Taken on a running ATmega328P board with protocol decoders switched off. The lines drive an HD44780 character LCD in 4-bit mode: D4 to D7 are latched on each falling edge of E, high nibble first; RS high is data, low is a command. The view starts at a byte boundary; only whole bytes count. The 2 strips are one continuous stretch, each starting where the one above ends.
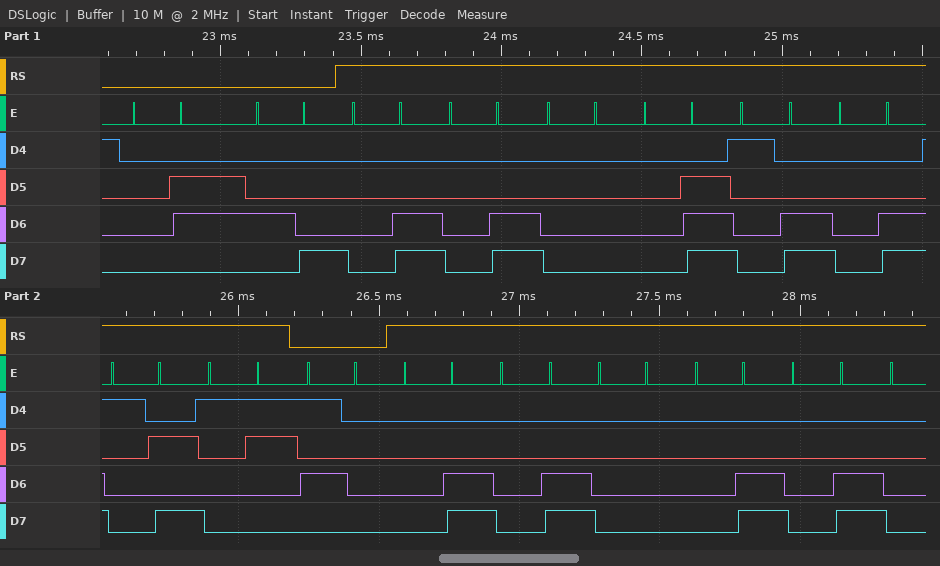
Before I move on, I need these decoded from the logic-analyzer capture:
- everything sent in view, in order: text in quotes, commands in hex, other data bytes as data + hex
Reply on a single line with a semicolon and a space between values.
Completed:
0x06 0x48 data 0C 0C 00 0E 1C 0C 1A 13 0x50 data 0C 0C 00 0C 0C
